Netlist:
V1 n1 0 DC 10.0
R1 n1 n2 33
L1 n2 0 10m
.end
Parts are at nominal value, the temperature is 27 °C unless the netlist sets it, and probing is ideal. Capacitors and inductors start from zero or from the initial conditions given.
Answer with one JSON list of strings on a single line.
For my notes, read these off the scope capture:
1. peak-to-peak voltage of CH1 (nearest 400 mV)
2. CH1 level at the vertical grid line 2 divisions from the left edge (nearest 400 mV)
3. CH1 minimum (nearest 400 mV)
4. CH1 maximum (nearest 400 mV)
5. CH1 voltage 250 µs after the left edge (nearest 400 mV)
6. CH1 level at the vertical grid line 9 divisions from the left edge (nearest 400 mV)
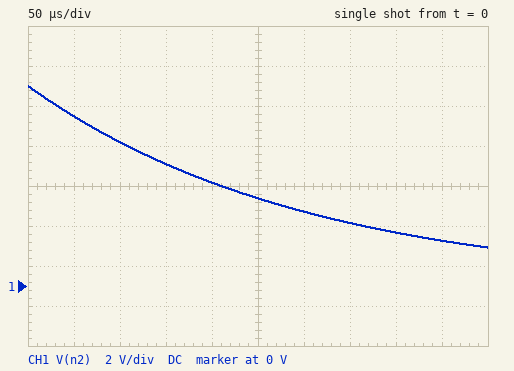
["8.0 V", "7.2 V", "2.0 V", "10.0 V", "4.4 V", "2.4 V"]
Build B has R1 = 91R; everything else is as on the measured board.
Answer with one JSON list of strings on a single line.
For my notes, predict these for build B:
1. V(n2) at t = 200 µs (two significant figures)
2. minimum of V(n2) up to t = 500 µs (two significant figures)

["1.6 V", "110 mV"]
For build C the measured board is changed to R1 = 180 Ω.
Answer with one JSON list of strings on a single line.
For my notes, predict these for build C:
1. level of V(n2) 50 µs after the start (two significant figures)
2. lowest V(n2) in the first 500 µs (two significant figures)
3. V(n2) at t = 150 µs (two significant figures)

["4.1 V", "1.2 mV", "670 mV"]
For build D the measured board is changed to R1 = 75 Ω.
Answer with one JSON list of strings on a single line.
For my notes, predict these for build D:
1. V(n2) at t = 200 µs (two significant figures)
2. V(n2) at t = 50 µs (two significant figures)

["2.2 V", "6.9 V"]
